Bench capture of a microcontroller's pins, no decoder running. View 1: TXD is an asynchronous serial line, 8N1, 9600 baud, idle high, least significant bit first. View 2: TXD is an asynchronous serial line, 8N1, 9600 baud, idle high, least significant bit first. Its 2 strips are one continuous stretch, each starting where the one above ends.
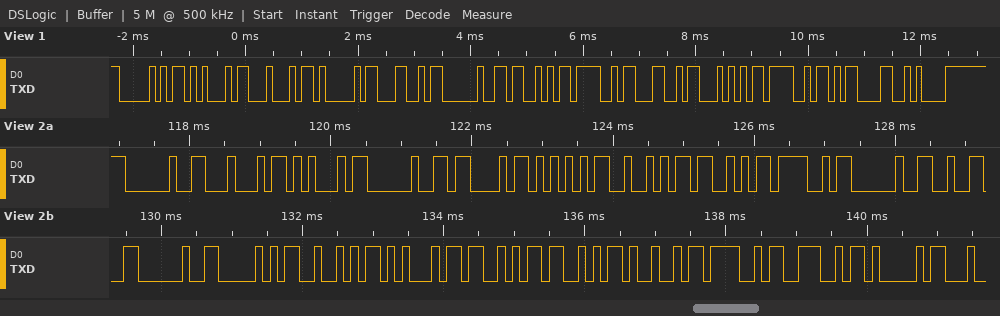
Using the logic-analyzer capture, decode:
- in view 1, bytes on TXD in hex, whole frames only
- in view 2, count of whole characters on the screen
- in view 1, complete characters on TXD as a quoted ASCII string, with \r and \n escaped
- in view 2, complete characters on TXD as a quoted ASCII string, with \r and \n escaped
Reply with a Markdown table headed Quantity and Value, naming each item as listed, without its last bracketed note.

| Quantity | Value |
|---|---|
| in view 1, bytes on TXD in hex, whole frames only | 50 45 44 41 4C 20 53 4F 4C 54 4F 0D 0A |
| in view 2, count of whole characters on the screen | 21 |
| in view 1, complete characters on TXD as a quoted ASCII string, with \r and \n escaped | "PEDAL SOLTO\r\n" |
| in view 2, complete characters on TXD as a quoted ASCII string, with \r and \n escaped | " DE CURSO 2 PRESSIONA" |
